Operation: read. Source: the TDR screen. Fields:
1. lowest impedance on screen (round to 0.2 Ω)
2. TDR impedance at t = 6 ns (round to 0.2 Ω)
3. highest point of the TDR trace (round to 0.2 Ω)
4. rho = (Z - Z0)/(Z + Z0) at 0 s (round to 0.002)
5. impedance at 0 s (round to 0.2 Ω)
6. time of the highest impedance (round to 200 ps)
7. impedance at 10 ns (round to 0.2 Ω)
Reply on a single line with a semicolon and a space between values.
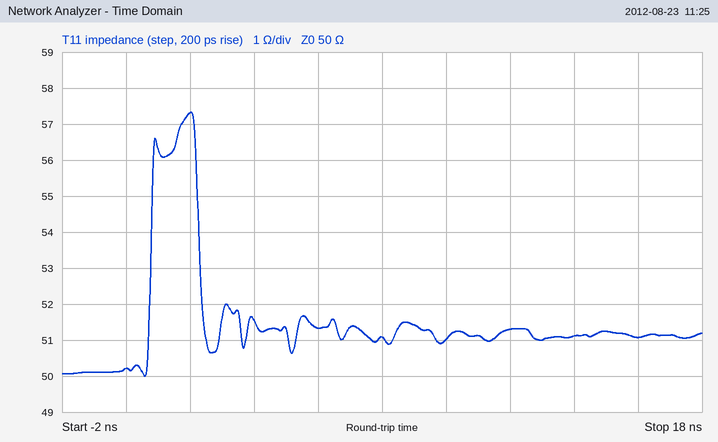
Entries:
50.0 Ω; 51.4 Ω; 57.4 Ω; +0.002; 50.2 Ω; 2.0 ns; 51.0 Ω
